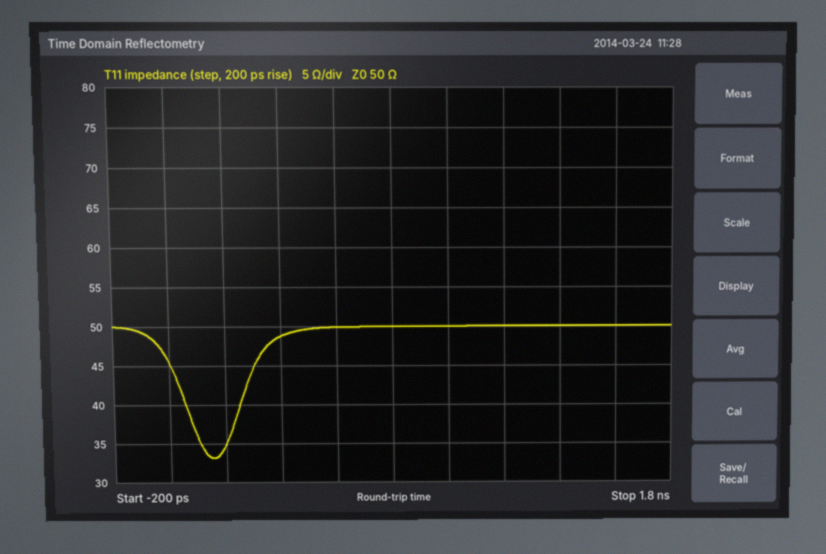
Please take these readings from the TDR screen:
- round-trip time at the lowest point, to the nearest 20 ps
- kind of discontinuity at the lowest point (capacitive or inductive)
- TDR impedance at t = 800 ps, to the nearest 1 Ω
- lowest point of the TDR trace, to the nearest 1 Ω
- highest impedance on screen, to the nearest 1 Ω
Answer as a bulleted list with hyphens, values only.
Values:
- 160 ps
- capacitive
- 50 Ω
- 33 Ω
- 50 Ω
